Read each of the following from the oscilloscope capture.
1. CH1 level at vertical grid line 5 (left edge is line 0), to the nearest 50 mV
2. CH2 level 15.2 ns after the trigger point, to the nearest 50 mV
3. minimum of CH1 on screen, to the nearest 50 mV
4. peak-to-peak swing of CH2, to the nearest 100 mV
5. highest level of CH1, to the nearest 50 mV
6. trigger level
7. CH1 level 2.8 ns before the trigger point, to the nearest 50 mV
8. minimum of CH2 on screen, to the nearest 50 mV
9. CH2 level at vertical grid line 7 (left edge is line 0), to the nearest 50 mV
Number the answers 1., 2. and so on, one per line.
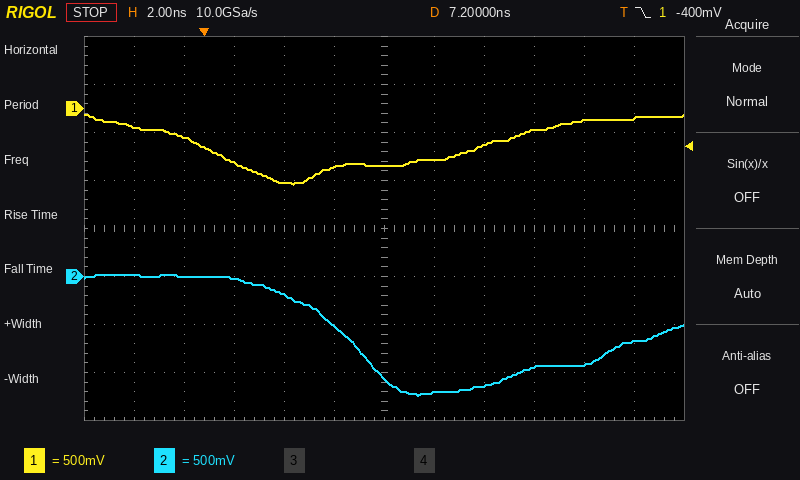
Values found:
1. -600 mV
2. -900 mV
3. -800 mV
4. 1.30 V
5. -50 mV
6. -400 mV
7. -200 mV
8. -1.25 V
9. -1.20 V
